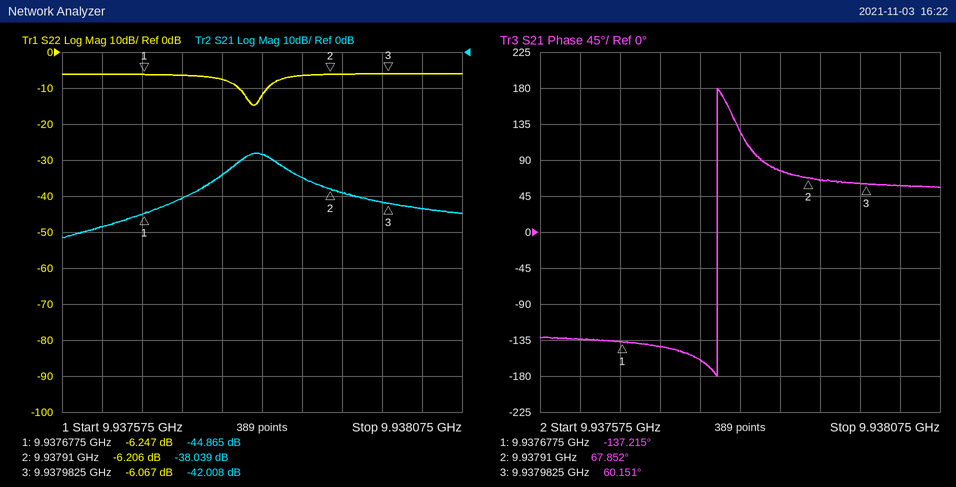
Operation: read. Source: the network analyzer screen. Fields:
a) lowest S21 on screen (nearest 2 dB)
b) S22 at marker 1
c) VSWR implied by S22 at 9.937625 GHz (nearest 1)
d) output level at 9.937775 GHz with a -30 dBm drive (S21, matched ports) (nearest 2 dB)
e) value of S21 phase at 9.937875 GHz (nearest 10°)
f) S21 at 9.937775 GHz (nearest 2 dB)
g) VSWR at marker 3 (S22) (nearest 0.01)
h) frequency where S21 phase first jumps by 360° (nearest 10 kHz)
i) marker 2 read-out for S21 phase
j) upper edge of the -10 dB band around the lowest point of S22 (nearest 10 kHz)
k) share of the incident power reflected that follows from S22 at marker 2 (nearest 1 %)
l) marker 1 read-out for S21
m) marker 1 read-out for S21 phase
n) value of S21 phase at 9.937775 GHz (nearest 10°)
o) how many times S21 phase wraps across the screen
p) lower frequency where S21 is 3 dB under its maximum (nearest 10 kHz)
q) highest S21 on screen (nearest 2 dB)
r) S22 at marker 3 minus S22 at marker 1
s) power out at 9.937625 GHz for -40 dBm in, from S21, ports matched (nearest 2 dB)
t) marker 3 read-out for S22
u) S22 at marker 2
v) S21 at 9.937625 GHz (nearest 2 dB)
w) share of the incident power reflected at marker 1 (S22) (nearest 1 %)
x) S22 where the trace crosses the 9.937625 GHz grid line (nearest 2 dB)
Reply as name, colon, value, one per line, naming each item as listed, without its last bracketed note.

lowest S21 on screen: -52 dB
S22 at marker 1: -6.247 dB
VSWR implied by S22 at 9.937625 GHz: 3
output level at 9.937775 GHz with a -30 dBm drive (S21, matched ports): -64 dBm
value of S21 phase at 9.937875 GHz: 80°
S21 at 9.937775 GHz: -34 dB
VSWR at marker 3 (S22): 2.98
frequency where S21 phase first jumps by 360°: 9.93780 GHz
marker 2 read-out for S21 phase: 67.852°
upper edge of the -10 dB band around the lowest point of S22: 9.93783 GHz
share of the incident power reflected that follows from S22 at marker 2: 24 %
marker 1 read-out for S21: -44.865 dB
marker 1 read-out for S21 phase: -137.215°
value of S21 phase at 9.937775 GHz: -160°
how many times S21 phase wraps across the screen: 1
lower frequency where S21 is 3 dB under its maximum: 9.93779 GHz
highest S21 on screen: -28 dB
S22 at marker 3 minus S22 at marker 1: 0.180 dB
power out at 9.937625 GHz for -40 dBm in, from S21, ports matched: -88 dBm
marker 3 read-out for S22: -6.067 dB
S22 at marker 2: -6.206 dB
S21 at 9.937625 GHz: -48 dB
share of the incident power reflected at marker 1 (S22): 24 %
S22 where the trace crosses the 9.937625 GHz grid line: -6 dB
